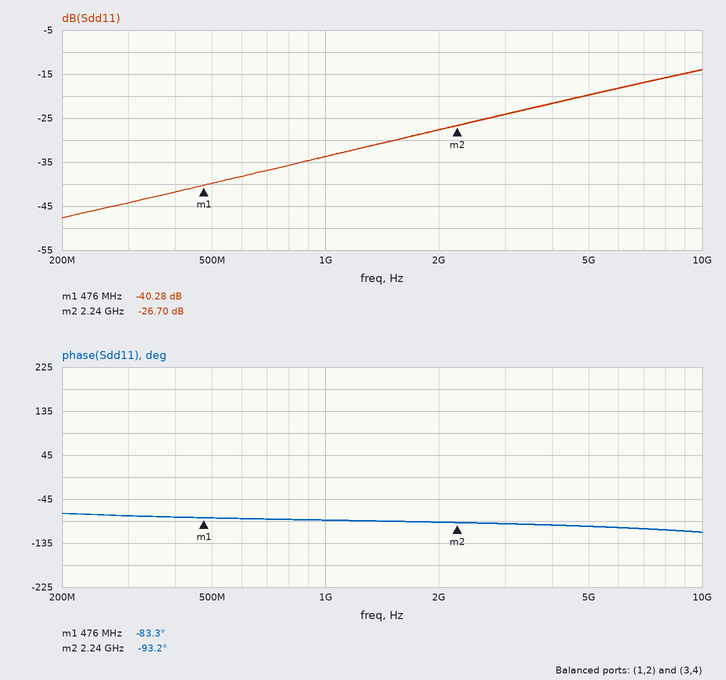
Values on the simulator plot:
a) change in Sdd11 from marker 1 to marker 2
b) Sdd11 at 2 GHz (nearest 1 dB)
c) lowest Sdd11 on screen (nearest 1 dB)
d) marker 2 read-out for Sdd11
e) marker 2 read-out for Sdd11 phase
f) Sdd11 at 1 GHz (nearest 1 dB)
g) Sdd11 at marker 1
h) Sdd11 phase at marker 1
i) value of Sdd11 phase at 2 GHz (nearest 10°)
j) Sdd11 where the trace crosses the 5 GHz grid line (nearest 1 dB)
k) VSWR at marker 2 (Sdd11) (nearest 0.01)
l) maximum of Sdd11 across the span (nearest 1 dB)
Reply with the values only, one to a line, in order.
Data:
13.58 dB
-28 dB
-48 dB
-26.70 dB
-93.2°
-34 dB
-40.28 dB
-83.3°
-90°
-20 dB
1.10
-14 dB
